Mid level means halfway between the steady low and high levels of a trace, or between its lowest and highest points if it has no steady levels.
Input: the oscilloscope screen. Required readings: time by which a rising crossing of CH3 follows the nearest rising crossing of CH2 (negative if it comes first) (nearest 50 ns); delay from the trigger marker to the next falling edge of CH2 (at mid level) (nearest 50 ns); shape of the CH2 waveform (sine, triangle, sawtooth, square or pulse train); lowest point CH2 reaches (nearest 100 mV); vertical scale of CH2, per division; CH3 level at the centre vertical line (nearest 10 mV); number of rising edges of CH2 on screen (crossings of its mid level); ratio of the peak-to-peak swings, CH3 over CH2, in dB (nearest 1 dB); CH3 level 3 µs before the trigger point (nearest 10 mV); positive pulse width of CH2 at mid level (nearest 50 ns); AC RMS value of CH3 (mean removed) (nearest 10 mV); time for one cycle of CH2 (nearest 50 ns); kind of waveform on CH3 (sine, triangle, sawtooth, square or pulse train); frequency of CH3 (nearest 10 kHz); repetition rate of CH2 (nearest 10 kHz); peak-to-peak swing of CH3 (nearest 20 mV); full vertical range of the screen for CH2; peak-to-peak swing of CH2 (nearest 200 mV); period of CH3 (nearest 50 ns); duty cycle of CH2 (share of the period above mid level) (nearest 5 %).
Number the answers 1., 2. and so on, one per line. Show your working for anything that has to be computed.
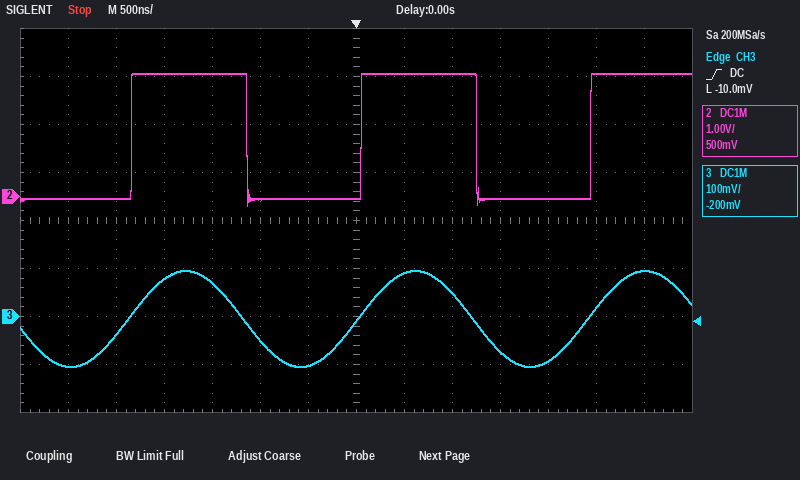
1. -50 ns
2. 1.25 µs
3. square
4. -200 mV
5. 1 V
6. -10 mV
7. 3
8. 20 log10(200 mV / 2.8 V) ≈ -23 dB
9. -100 mV
10. 1.20 µs
11. 200 mV / (2√2) ≈ 70.7 mV, so 70 mV to the nearest 10 mV
12. 2.40 µs
13. sine
14. 1 / 2.40 µs ≈ 417 kHz, so 420 kHz to the nearest 10 kHz
15. 1 / 2.40 µs ≈ 417 kHz, so 420 kHz to the nearest 10 kHz
16. 200 mV
17. 8 V
18. 2.8 V
19. 2.40 µs
20. 1.20 µs / 2.40 µs ≈ 50 %
